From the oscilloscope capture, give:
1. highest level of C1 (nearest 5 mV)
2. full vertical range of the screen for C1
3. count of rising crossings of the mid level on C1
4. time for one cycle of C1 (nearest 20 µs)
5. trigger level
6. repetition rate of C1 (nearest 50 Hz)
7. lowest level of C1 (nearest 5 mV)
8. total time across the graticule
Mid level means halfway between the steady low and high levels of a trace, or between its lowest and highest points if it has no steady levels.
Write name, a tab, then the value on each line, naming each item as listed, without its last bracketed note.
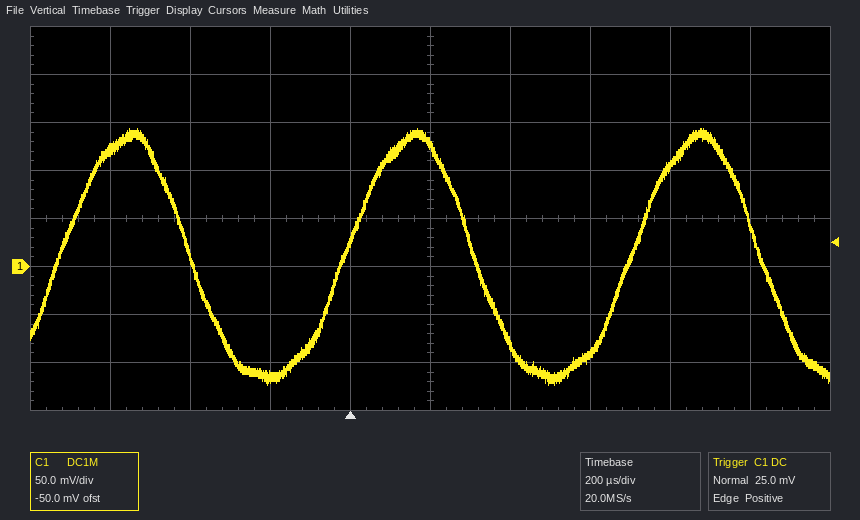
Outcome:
highest level of C1	145 mV
full vertical range of the screen for C1	400 mV
count of rising crossings of the mid level on C1	3
time for one cycle of C1	720 µs
trigger level	25.0 mV
repetition rate of C1	1.40 kHz
lowest level of C1	-125 mV
total time across the graticule	2 ms
